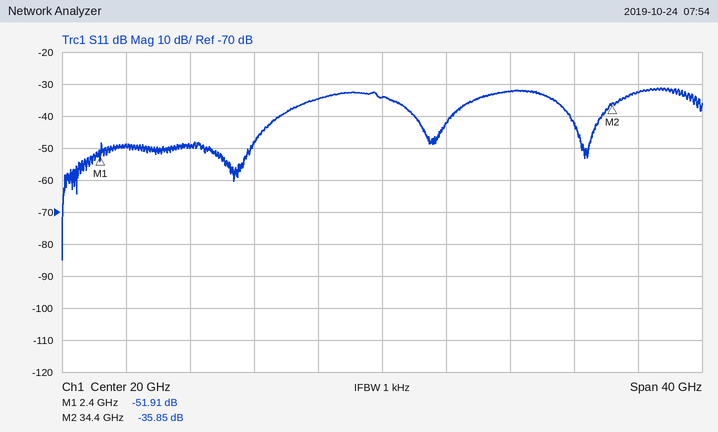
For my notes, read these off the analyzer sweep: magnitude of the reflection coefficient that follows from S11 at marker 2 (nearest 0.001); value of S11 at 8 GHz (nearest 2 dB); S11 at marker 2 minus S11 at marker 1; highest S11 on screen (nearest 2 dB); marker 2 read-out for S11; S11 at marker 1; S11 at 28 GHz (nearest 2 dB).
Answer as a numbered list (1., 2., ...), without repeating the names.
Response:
1. 0.016
2. -50 dB
3. 16.06 dB
4. -32 dB
5. -35.85 dB
6. -51.91 dB
7. -32 dB
